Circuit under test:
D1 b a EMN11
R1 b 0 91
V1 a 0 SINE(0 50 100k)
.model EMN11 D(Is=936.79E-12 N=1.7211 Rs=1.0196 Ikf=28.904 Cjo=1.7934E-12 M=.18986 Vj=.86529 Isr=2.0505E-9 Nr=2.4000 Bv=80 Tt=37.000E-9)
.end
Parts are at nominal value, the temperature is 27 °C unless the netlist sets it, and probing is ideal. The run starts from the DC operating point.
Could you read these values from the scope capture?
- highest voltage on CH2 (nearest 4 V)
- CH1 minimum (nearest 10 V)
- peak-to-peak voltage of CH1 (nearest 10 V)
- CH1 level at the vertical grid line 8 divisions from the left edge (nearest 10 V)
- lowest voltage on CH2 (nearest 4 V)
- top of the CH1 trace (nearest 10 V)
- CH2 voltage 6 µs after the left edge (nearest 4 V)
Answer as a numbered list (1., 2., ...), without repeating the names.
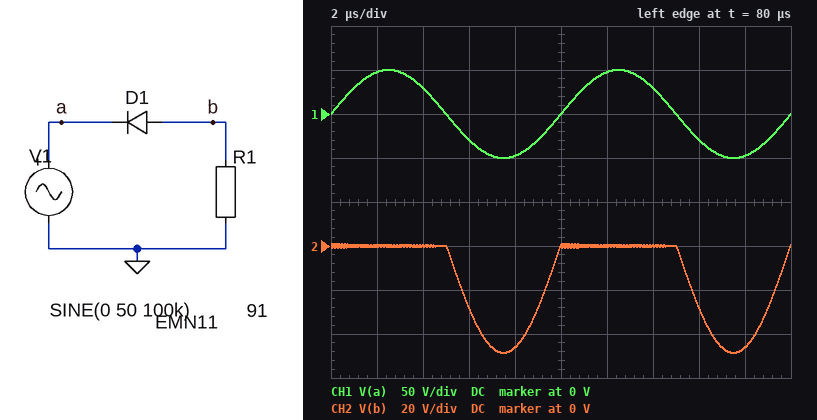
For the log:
1. 0 V
2. -50 V
3. 100 V
4. -30 V
5. -48 V
6. 50 V
7. -28 V
